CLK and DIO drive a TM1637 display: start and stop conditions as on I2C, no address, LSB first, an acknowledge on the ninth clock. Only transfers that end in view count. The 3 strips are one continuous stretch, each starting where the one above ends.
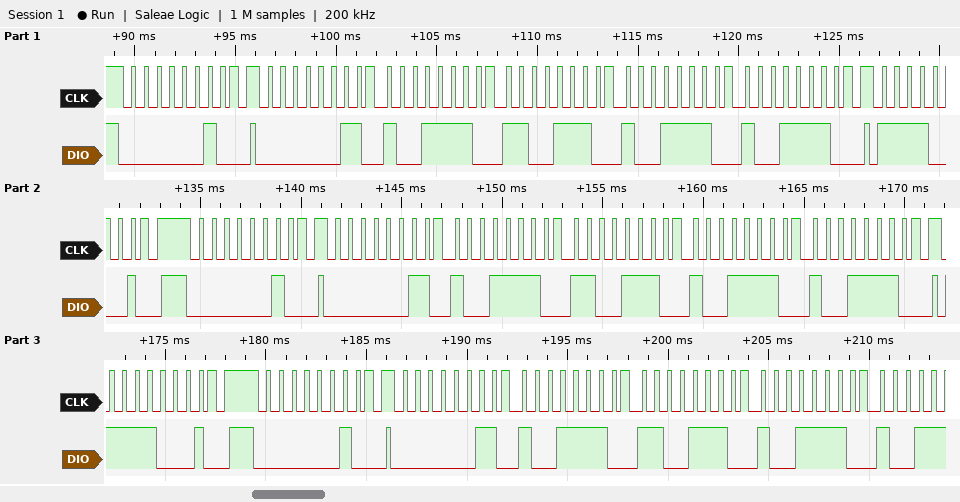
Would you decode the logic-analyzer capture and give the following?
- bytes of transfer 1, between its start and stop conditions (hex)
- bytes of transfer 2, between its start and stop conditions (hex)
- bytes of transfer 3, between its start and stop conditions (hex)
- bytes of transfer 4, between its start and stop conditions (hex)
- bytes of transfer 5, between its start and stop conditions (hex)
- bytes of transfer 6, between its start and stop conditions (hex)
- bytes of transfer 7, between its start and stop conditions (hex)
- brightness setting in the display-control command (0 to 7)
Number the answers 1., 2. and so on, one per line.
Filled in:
1. 40
2. C0 79 73 79 79
3. 8F
4. 40
5. C0 79 73 79 79
6. 8F
7. 40
8. 7
